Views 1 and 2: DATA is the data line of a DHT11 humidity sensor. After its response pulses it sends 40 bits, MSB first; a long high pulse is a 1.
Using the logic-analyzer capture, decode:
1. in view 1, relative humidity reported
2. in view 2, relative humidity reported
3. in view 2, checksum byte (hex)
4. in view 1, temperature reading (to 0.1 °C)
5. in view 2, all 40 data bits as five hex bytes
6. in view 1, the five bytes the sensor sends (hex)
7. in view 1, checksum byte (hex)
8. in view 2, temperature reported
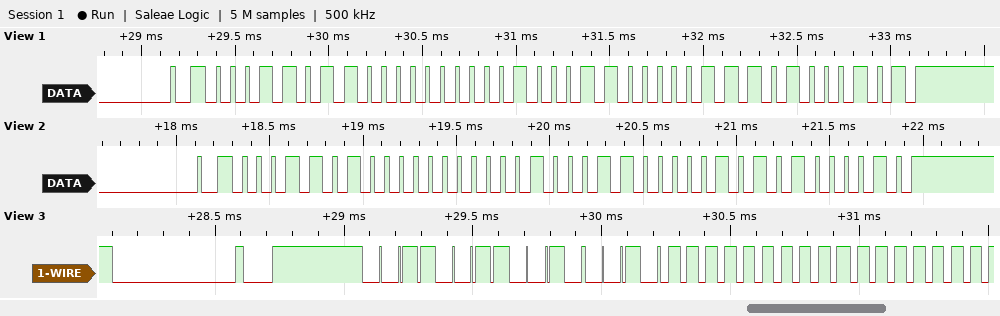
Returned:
27 %
26 %
0x42
35.7 °C
1A 00 23 05 42
1B 00 23 07 45
0x45
35.5 °C
